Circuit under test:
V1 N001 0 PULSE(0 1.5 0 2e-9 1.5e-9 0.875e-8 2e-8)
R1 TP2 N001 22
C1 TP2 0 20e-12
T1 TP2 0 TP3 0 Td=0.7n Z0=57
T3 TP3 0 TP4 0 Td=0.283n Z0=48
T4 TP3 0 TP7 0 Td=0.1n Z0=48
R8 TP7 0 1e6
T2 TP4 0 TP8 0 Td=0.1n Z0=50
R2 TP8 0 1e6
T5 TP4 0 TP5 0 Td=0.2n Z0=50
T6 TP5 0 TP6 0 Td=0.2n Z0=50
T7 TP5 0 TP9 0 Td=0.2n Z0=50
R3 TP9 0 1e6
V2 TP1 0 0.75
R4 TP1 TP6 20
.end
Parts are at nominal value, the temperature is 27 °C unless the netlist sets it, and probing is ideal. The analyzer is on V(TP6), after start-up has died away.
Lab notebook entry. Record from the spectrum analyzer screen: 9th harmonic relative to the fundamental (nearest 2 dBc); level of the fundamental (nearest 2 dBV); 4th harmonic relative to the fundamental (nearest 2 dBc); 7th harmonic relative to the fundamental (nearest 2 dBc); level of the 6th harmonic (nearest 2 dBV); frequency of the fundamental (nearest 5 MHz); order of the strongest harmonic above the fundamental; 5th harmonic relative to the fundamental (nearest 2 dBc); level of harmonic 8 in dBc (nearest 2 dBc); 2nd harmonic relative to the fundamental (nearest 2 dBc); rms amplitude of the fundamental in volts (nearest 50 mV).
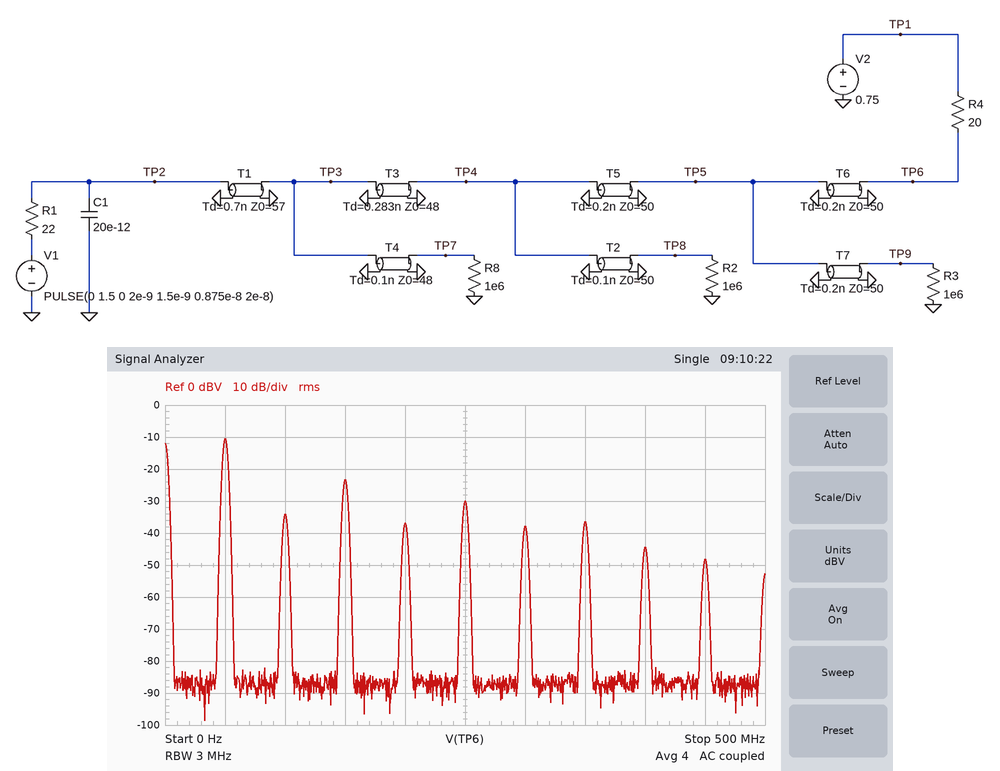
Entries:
-38 dBc
-10 dBV
-26 dBc
-26 dBc
-38 dBV
50 MHz
3
-20 dBc
-34 dBc
-24 dBc
300 mV
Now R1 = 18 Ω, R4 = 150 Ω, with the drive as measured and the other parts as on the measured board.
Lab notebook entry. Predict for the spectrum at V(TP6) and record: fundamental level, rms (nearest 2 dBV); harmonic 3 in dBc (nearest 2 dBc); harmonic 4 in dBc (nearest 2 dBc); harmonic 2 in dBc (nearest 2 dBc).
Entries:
-4 dBV
-8 dBc
-22 dBc
-20 dBc
